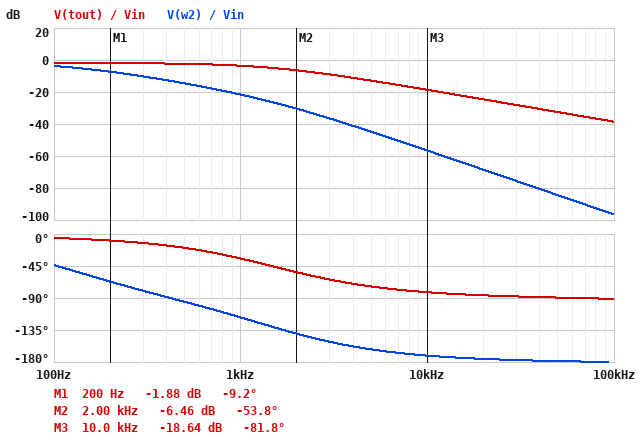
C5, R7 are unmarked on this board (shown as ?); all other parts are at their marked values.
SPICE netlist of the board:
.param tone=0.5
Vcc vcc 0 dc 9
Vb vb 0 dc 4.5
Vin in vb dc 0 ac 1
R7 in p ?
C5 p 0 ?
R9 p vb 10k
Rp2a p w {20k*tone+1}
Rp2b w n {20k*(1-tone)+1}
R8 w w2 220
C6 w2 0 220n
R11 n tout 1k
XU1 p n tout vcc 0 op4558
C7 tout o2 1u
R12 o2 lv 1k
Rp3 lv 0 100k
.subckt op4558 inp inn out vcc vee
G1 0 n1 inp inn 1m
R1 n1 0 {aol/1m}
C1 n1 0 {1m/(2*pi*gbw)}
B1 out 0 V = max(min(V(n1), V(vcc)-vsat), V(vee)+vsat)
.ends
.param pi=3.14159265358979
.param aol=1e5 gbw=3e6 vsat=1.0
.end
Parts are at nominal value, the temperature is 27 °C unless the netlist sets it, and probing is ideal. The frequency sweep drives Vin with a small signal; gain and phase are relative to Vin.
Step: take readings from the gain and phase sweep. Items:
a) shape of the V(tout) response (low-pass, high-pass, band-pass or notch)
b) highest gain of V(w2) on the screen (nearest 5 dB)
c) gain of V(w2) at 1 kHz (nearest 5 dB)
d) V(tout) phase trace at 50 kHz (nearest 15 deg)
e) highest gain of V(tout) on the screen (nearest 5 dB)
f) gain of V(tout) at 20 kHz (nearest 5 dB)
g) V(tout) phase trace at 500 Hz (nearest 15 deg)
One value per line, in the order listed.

low-pass
-5 dB
-20 dB
-90 deg
0 dB
-25 dB
-15 deg
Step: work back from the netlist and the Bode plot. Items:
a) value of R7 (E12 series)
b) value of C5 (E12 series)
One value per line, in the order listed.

1.8 kΩ
82 nF
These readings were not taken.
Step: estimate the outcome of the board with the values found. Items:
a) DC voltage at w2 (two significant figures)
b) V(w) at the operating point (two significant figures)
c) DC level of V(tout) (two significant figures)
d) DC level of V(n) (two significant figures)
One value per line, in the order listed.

4.5 V
4.5 V
4.5 V
4.5 V
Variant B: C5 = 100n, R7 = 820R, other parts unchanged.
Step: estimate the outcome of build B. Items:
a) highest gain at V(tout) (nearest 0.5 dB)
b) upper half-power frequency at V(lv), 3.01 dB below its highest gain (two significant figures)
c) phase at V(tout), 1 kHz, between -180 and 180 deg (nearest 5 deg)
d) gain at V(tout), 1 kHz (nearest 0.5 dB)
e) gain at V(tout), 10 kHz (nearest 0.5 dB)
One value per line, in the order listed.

-0.5 dB
2.3 kHz
-25 deg
-1.5 dB
-13.5 dB
